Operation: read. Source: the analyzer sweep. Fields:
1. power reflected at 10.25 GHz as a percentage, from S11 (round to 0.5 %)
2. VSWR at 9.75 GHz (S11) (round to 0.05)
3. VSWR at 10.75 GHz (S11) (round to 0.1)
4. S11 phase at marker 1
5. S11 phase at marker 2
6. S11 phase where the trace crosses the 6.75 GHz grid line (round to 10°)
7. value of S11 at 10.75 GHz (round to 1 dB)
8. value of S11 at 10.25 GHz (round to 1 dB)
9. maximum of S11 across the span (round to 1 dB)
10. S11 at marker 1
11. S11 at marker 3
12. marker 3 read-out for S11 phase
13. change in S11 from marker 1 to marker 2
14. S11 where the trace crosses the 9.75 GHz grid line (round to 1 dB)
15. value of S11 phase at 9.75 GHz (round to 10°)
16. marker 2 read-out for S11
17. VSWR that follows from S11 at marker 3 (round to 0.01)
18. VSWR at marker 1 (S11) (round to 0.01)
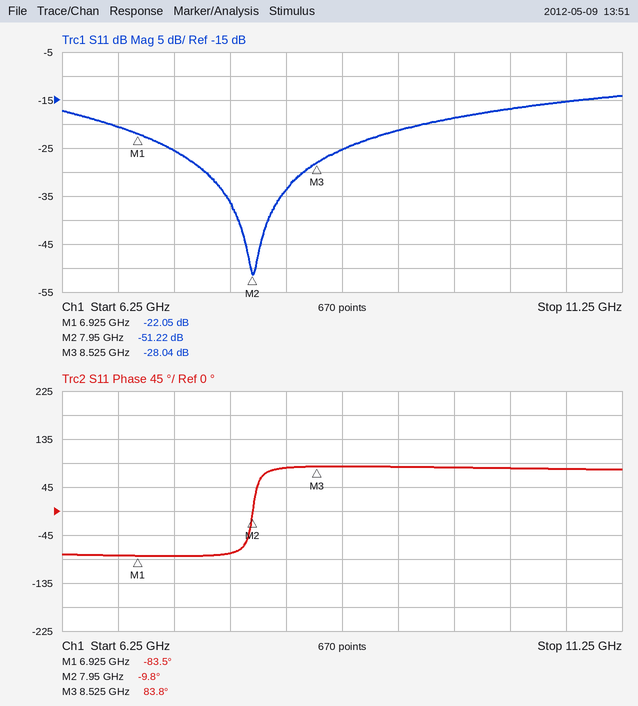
2.0 %
1.25
1.4
-83.5°
-9.8°
-80°
-15 dB
-17 dB
-14 dB
-22.05 dB
-28.04 dB
83.8°
-29.17 dB
-19 dB
80°
-51.22 dB
1.08
1.17
